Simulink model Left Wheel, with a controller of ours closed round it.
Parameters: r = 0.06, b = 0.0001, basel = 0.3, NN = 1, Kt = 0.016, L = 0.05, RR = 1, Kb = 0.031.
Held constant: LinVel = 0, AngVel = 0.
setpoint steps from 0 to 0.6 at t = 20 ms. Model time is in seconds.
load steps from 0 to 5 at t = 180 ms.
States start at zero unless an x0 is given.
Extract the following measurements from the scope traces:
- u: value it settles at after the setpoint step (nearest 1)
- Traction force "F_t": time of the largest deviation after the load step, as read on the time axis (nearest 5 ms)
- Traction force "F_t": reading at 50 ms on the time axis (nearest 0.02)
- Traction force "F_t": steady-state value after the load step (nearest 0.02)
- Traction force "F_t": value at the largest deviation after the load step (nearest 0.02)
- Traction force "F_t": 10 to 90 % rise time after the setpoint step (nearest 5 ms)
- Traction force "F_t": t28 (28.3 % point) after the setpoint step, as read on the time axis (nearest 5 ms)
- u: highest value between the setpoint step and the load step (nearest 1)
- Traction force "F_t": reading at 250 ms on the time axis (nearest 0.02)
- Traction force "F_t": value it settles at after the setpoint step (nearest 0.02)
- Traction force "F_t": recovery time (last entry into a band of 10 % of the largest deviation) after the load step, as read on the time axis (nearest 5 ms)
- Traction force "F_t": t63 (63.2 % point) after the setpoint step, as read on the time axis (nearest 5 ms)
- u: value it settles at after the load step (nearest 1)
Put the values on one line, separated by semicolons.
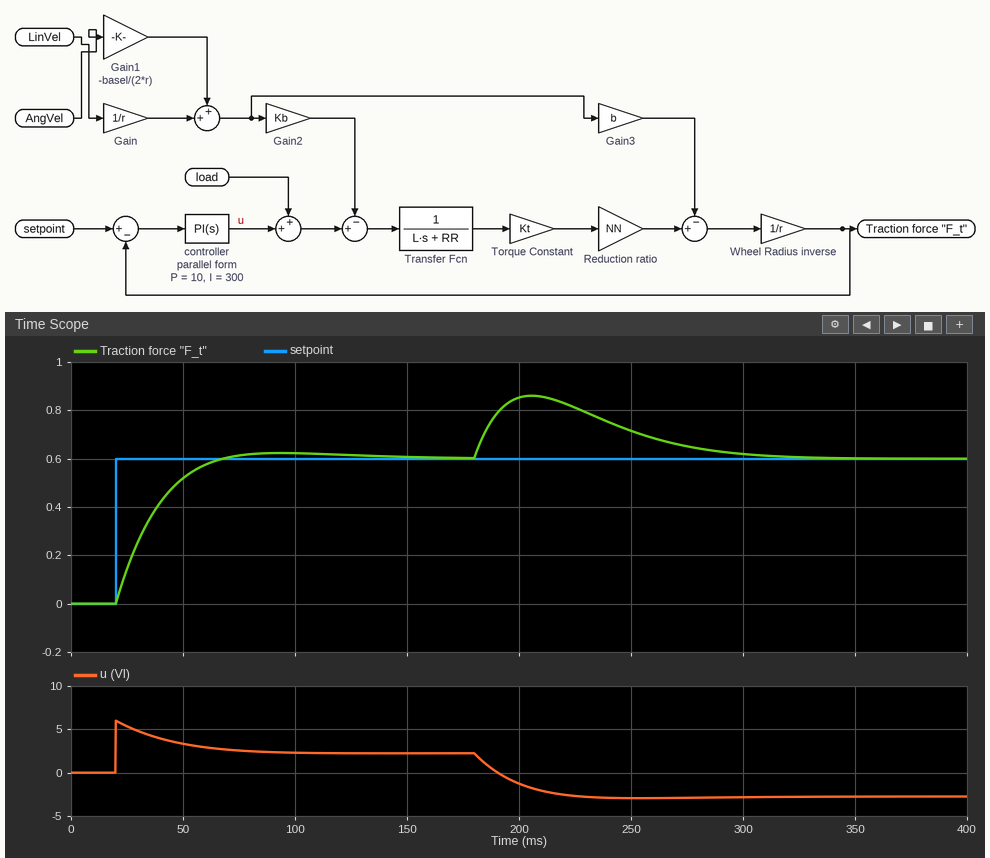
2; 205 ms; 0.52; 0.60; 0.86; 30 ms; 25 ms; 6; 0.72; 0.60; 295 ms; 35 ms; -3
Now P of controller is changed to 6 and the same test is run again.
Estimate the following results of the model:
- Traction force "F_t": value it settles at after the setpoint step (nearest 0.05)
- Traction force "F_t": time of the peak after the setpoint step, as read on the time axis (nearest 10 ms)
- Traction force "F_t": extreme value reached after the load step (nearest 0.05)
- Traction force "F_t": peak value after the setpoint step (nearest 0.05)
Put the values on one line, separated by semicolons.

0.60; 90 ms; 0.90; 0.65
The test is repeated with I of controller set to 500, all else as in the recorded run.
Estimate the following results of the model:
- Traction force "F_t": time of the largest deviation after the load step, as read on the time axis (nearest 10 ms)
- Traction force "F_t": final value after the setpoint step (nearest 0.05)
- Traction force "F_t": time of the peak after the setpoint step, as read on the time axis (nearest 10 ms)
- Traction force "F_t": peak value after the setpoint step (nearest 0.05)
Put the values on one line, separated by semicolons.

200 ms; 0.60; 70 ms; 0.65
